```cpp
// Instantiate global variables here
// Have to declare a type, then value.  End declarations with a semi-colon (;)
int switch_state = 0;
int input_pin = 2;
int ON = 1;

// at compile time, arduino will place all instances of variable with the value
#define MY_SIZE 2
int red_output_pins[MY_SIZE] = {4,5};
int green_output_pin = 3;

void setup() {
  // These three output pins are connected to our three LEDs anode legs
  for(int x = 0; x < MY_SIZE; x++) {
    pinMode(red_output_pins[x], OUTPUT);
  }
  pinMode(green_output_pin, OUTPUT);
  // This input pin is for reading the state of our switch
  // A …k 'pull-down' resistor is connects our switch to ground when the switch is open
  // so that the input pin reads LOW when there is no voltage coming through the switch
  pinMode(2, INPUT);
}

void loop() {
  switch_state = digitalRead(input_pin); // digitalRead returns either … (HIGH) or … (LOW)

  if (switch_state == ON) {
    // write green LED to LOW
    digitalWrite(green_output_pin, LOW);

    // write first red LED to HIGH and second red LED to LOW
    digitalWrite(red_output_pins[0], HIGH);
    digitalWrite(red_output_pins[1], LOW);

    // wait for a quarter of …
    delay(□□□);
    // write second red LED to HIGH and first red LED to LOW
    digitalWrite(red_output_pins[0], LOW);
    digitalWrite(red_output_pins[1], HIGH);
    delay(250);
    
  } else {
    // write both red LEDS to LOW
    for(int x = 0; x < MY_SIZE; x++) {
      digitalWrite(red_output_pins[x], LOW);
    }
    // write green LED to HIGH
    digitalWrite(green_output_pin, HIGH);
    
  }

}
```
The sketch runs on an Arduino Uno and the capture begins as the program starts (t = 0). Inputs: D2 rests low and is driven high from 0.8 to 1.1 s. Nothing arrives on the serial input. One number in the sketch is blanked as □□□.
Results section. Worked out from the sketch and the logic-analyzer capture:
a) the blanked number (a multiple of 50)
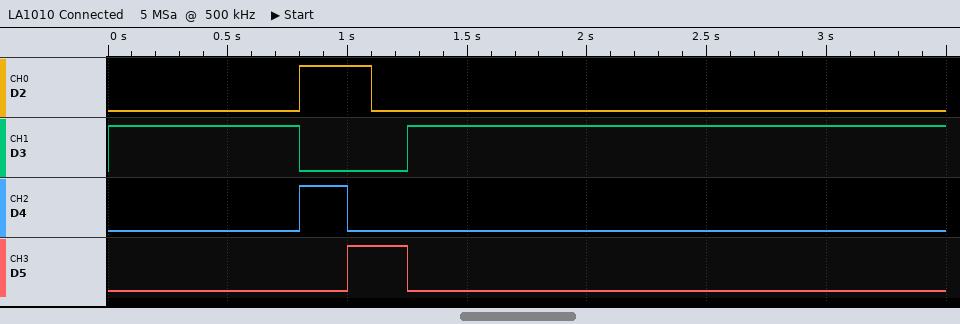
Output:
200
